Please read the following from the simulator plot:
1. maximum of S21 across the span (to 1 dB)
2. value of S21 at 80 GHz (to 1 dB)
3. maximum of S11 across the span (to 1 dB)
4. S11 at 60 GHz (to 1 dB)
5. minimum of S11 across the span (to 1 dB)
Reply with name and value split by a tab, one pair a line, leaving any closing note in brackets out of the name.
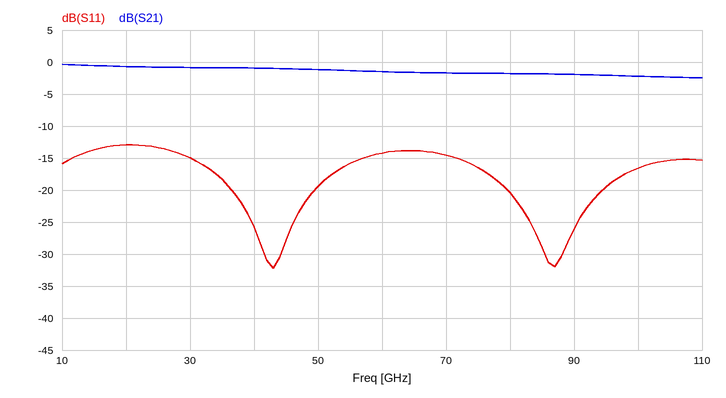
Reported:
maximum of S21 across the span	0 dB
value of S21 at 80 GHz	-2 dB
maximum of S11 across the span	-13 dB
S11 at 60 GHz	-14 dB
minimum of S11 across the span	-32 dB
